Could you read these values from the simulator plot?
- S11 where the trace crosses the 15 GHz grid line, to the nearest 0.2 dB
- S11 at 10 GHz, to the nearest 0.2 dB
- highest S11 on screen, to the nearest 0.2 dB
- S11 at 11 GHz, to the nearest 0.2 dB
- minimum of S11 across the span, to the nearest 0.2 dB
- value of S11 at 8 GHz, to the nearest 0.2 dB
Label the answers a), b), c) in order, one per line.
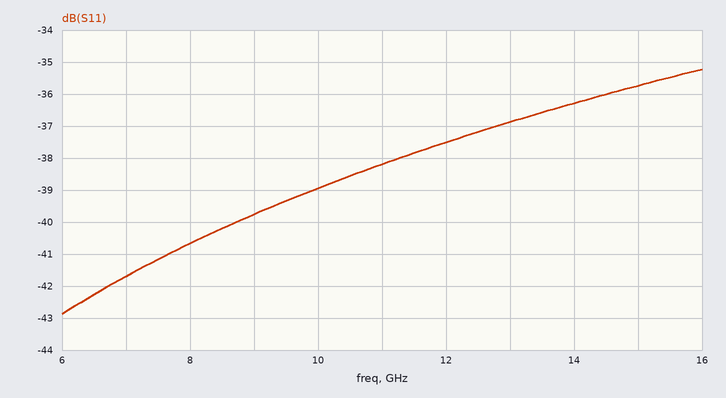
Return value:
a) -35.8 dB
b) -39.0 dB
c) -35.2 dB
d) -38.2 dB
e) -42.8 dB
f) -40.6 dB
